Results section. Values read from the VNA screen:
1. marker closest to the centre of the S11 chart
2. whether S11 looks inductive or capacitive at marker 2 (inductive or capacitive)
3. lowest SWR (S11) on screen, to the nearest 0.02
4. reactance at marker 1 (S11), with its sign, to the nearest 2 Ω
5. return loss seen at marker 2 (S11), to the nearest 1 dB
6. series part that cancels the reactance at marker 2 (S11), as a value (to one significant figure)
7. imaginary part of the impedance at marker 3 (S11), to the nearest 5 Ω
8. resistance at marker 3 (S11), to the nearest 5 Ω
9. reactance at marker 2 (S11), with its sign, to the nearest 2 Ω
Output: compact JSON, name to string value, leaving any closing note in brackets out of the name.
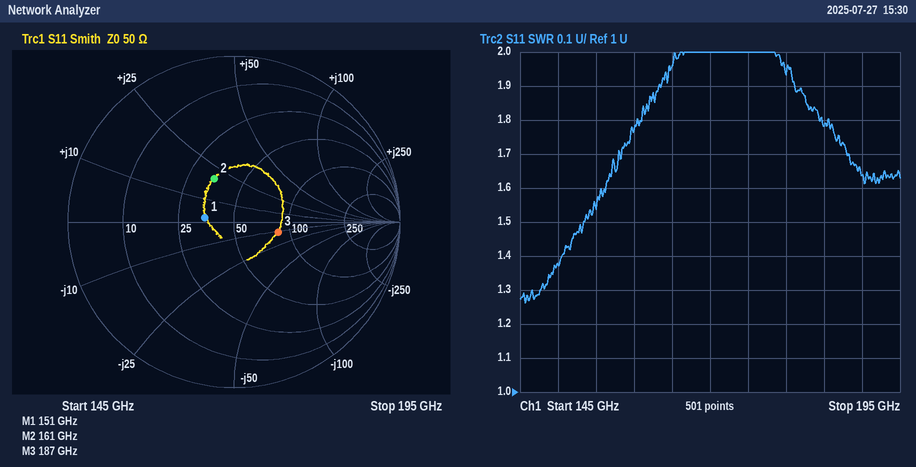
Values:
{"marker closest to the centre of the S11 chart": "marker 1", "whether S11 looks inductive or capacitive at marker 2": "inductive", "lowest SWR (S11) on screen, to the nearest 0.02": "1.26", "reactance at marker 1 (S11), with its sign, to the nearest 2 Ω": "+2 Ω", "return loss seen at marker 2 (S11), to the nearest 1 dB": "11 dB", "series part that cancels the reactance at marker 2 (S11), as a value": "50 fF", "imaginary part of the impedance at marker 3 (S11), to the nearest 5 Ω": "-10 Ω", "resistance at marker 3 (S11), to the nearest 5 Ω": "85 Ω", "reactance at marker 2 (S11), with its sign, to the nearest 2 Ω": "+20 Ω"}
